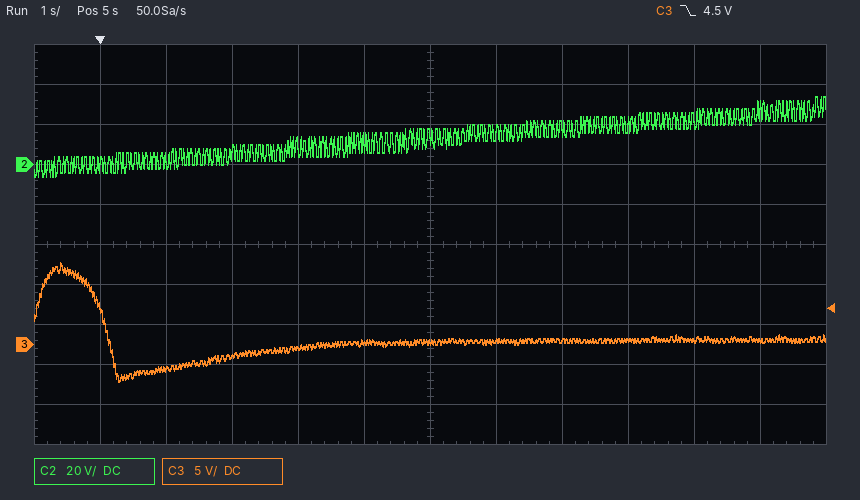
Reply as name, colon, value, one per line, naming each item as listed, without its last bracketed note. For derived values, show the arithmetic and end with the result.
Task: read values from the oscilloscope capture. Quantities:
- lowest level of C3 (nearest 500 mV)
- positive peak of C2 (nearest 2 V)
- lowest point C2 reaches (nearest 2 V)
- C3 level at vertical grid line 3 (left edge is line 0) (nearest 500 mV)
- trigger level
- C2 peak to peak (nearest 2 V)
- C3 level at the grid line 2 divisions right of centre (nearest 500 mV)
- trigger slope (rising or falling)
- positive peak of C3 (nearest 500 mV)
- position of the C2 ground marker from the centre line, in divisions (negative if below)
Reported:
lowest level of C3: -4.5 V
positive peak of C2: 34 V
lowest point C2 reaches: -6 V
C3 level at vertical grid line 3 (left edge is line 0): -1.5 V
trigger level: 4.5 V
C2 peak to peak: 34 V − (-6 V) = 40 V
C3 level at the grid line 2 divisions right of centre: 500 mV
trigger slope: falling
positive peak of C3: 10.0 V
position of the C2 ground marker from the centre line, in divisions: +2.0 div
